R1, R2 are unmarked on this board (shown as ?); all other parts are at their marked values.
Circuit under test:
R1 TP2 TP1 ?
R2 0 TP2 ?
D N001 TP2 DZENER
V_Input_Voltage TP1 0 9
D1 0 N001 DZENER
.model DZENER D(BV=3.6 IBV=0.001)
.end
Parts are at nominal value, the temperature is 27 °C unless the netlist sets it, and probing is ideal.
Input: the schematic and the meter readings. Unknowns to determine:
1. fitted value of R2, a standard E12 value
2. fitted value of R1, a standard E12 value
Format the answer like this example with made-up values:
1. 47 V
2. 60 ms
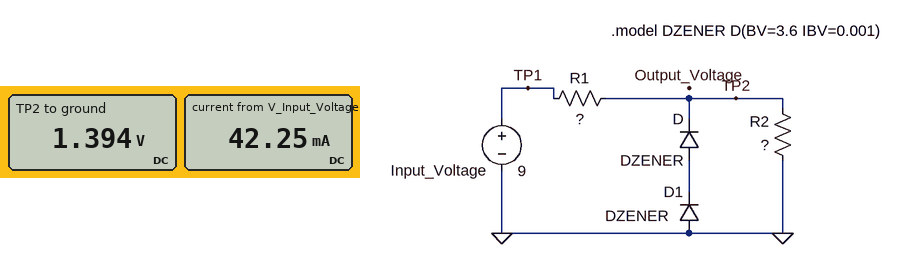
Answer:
1. 33 Ω
2. 180 Ω
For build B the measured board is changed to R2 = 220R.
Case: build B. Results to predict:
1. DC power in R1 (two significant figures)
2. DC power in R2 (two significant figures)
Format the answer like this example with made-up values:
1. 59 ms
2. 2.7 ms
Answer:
1. 91 mW
2. 110 mW
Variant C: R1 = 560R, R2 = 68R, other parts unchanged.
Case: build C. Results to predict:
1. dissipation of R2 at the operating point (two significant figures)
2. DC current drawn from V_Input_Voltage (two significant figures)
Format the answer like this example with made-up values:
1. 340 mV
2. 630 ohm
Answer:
1. 14 mW
2. 14 mA
